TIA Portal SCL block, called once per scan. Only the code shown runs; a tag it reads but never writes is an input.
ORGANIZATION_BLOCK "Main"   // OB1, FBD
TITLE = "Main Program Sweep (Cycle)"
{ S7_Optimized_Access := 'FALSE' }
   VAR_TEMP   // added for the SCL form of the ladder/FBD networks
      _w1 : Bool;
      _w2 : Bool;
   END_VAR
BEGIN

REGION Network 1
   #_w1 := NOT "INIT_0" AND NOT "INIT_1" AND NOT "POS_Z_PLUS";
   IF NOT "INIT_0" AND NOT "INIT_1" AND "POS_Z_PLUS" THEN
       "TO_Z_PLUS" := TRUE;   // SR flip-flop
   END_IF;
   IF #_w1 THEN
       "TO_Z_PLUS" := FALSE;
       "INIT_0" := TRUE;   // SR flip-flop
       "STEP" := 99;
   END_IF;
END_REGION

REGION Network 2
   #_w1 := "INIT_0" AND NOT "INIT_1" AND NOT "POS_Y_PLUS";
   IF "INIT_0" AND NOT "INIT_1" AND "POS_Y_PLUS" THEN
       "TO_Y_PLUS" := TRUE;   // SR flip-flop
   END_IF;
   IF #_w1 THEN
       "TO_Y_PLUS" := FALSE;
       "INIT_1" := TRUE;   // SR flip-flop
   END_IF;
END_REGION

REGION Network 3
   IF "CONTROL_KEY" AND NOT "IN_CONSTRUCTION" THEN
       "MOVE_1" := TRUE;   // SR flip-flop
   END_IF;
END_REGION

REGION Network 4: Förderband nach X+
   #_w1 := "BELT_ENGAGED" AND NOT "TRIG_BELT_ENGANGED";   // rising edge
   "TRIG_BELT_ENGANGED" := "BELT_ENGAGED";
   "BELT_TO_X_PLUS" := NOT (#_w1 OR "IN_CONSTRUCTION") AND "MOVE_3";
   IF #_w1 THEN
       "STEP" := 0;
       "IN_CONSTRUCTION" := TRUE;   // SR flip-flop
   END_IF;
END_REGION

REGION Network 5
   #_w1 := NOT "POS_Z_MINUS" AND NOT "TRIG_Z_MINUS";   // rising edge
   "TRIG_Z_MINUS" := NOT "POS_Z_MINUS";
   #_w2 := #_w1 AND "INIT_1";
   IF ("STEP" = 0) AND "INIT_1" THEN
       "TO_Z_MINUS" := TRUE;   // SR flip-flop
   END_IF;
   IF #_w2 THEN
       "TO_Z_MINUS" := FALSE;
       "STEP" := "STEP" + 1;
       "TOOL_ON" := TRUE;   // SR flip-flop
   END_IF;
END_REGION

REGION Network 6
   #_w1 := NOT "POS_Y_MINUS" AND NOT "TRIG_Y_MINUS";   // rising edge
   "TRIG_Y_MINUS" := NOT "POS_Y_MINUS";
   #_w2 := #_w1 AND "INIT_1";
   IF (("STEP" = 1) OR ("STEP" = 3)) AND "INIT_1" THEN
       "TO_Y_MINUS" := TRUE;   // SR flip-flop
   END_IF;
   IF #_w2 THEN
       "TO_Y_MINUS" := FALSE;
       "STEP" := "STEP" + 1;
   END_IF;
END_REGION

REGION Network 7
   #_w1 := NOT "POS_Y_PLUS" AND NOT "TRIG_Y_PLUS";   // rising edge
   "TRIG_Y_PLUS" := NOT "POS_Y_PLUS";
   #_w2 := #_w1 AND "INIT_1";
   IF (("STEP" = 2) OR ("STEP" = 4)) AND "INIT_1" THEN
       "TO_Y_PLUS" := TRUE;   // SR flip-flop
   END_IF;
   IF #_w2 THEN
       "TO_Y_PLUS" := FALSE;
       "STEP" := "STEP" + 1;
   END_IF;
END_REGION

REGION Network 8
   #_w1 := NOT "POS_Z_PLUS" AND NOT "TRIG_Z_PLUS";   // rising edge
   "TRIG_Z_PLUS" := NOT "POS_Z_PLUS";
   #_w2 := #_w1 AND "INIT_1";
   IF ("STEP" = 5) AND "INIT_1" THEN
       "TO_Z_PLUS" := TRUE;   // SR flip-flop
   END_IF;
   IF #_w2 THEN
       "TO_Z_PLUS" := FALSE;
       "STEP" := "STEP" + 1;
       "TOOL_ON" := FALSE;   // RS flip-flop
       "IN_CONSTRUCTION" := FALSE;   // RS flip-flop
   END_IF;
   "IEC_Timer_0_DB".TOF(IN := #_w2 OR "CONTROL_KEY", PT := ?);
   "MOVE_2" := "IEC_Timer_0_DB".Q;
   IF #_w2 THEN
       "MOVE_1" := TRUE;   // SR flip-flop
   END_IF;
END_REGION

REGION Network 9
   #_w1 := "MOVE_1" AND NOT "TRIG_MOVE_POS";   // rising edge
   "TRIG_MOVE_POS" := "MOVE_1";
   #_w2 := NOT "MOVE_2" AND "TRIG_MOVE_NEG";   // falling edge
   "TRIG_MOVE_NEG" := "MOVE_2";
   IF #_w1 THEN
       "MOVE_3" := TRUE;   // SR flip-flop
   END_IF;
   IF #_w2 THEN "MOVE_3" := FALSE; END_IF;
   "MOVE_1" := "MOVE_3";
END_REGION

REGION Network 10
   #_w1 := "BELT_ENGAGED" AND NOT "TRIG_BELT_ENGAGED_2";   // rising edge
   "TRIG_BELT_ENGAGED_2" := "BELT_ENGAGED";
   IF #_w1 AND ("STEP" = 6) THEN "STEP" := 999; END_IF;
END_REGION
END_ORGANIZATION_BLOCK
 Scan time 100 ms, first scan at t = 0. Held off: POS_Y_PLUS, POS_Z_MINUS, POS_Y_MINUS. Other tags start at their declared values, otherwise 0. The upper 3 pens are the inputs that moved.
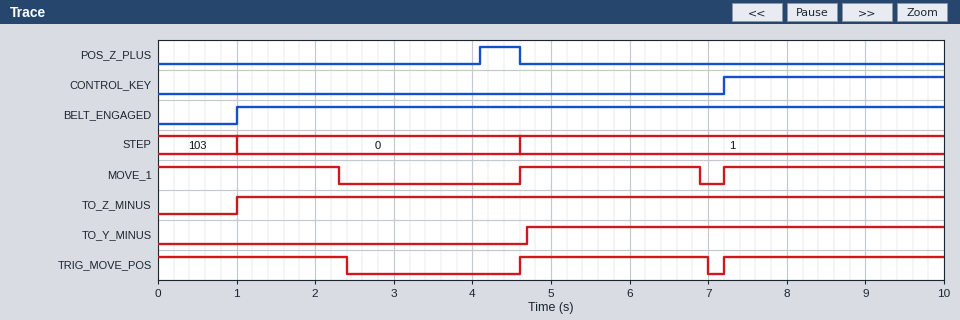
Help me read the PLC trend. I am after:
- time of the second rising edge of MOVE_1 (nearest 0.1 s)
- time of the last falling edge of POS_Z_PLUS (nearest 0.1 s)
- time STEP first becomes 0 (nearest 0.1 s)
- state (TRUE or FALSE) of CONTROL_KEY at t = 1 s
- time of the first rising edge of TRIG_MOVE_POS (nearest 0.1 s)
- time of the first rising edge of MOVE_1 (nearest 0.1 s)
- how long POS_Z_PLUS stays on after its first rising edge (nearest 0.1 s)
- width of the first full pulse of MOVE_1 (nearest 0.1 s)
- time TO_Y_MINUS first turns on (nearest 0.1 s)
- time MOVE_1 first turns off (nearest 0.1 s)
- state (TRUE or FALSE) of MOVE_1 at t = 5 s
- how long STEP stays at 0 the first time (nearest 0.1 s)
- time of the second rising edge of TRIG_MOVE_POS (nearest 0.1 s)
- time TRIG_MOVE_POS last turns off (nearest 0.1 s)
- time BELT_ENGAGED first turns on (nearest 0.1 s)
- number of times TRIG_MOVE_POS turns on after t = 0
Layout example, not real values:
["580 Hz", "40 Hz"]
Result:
["7.2 s", "4.6 s", "1.0 s", "FALSE", "4.6 s", "4.6 s", "0.5 s", "2.3 s", "4.7 s", "2.3 s", "TRUE", "3.6 s", "7.2 s", "7.0 s", "1.0 s", "2"]
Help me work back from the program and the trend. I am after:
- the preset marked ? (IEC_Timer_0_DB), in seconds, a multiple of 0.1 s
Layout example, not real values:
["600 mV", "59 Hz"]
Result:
["2.2 s"]
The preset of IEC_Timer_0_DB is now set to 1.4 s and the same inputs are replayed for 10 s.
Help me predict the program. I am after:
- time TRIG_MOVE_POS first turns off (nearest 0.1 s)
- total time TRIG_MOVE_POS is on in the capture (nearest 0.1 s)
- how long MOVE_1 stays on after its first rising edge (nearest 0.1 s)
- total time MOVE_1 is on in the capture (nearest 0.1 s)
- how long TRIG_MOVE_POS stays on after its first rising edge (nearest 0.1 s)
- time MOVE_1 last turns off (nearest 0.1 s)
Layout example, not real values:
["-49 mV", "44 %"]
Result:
["1.6 s", "6.0 s", "1.5 s", "5.8 s", "1.6 s", "6.1 s"]
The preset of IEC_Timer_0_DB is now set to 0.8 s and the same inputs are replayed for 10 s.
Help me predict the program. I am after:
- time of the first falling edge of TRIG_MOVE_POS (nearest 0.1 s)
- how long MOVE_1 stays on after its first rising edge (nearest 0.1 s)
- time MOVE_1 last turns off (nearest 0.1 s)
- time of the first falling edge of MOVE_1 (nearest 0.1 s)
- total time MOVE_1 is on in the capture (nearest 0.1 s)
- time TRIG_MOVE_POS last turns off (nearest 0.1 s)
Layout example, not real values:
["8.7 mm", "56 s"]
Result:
["1.0 s", "0.9 s", "5.5 s", "0.9 s", "4.6 s", "5.6 s"]
